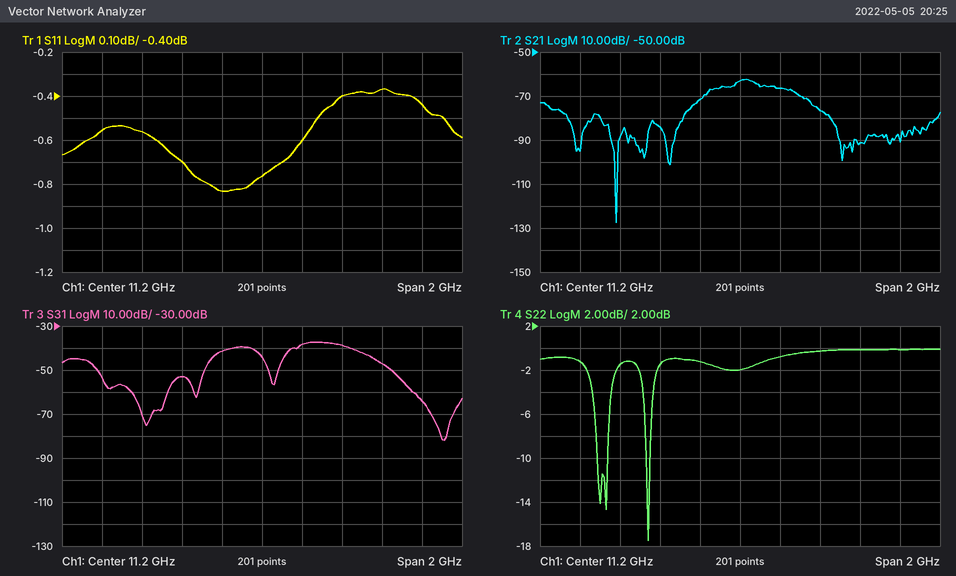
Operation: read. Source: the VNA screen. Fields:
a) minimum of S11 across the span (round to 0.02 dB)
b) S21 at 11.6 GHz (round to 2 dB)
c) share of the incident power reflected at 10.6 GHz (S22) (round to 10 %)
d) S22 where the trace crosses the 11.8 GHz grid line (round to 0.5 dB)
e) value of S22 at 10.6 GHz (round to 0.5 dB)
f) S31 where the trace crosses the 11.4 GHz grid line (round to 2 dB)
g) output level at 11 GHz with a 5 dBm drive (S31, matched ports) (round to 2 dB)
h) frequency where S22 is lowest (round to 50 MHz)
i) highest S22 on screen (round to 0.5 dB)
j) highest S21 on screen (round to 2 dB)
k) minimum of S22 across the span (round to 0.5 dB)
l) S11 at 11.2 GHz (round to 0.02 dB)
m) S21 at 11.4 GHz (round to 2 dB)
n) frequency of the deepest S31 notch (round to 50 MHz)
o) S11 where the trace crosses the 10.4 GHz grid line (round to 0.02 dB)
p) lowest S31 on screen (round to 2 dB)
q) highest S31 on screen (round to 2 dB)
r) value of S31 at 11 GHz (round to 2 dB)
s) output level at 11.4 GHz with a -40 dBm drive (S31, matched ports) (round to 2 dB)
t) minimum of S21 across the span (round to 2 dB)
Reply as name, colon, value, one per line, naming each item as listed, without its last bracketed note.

minimum of S11 across the span: -0.84 dB
S21 at 11.6 GHz: -76 dB
share of the incident power reflected at 10.6 GHz (S22): 70 %
S22 where the trace crosses the 11.8 GHz grid line: 0.0 dB
value of S22 at 10.6 GHz: -1.5 dB
S31 where the trace crosses the 11.4 GHz grid line: -38 dB
output level at 11 GHz with a 5 dBm drive (S31, matched ports): -36 dBm
frequency where S22 is lowest: 10.75 GHz
highest S22 on screen: 0.0 dB
highest S21 on screen: -62 dB
minimum of S22 across the span: -17.5 dB
S11 at 11.2 GHz: -0.76 dB
S21 at 11.4 GHz: -66 dB
frequency of the deepest S31 notch: 12.10 GHz
S11 where the trace crosses the 10.4 GHz grid line: -0.56 dB
lowest S31 on screen: -82 dB
highest S31 on screen: -38 dB
value of S31 at 11 GHz: -42 dB
output level at 11.4 GHz with a -40 dBm drive (S31, matched ports): -78 dBm
minimum of S21 across the span: -128 dB
